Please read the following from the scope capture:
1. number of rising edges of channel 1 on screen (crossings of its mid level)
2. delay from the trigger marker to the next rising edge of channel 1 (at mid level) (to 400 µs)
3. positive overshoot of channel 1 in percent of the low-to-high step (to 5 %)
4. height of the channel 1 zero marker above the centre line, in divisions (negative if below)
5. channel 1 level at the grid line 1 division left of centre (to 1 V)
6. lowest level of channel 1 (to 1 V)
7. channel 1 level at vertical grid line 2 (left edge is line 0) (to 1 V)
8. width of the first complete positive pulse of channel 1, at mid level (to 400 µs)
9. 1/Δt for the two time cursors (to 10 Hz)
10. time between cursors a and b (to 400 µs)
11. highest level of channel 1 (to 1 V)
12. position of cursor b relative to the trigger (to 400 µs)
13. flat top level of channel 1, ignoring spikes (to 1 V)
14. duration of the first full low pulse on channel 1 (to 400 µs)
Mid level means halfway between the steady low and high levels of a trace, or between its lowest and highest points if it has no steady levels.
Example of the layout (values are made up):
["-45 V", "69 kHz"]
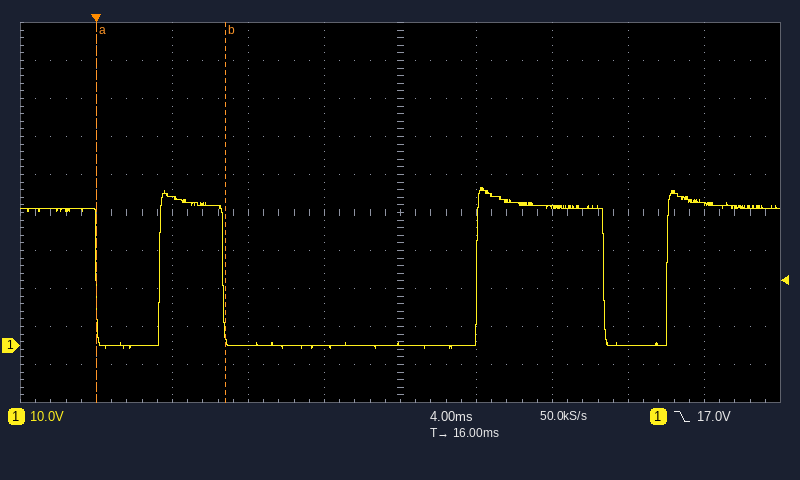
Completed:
["3", "3.2 ms", "15 %", "-3.5 div", "0 V", "-1 V", "39 V", "3.2 ms", "150 Hz", "6.8 ms", "42 V", "+6.8 ms", "36 V", "3.2 ms"]
